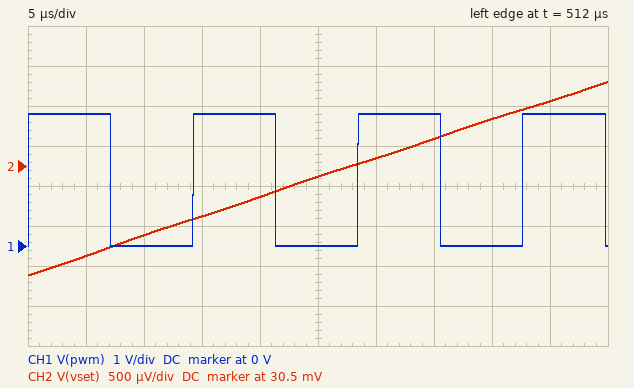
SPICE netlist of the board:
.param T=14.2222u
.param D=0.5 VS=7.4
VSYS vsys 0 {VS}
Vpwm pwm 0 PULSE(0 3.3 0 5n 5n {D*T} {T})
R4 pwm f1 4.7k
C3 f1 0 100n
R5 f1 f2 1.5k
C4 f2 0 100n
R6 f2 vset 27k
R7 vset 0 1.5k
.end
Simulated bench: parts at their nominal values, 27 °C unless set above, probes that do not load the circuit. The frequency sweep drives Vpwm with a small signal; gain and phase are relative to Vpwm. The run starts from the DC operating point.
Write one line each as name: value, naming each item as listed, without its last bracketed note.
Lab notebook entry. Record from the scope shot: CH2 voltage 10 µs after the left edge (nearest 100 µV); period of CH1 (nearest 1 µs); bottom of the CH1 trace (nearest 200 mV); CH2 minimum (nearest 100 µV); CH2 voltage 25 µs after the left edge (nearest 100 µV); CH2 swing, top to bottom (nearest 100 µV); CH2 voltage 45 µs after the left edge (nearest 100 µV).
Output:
CH2 voltage 10 µs after the left edge: 29.6 mV
period of CH1: 14 µs
bottom of the CH1 trace: 0 V
CH2 minimum: 29.1 mV
CH2 voltage 25 µs after the left edge: 30.4 mV
CH2 swing, top to bottom: 2.4 mV
CH2 voltage 45 µs after the left edge: 31.3 mV
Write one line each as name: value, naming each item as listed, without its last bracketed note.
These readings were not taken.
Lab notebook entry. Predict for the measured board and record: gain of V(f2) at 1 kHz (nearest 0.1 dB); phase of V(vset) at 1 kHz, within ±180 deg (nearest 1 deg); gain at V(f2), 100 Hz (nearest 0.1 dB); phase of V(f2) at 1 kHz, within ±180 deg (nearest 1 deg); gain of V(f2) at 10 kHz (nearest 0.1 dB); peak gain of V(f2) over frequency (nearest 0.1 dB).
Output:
gain of V(f2) at 1 kHz: -17.1 dB
phase of V(vset) at 1 kHz, within ±180 deg: -103 deg
gain at V(f2), 100 Hz: -2.8 dB
phase of V(f2) at 1 kHz, within ±180 deg: -103 deg
gain of V(f2) at 10 kHz: -49.1 dB
peak gain of V(f2) over frequency: -1.7 dB
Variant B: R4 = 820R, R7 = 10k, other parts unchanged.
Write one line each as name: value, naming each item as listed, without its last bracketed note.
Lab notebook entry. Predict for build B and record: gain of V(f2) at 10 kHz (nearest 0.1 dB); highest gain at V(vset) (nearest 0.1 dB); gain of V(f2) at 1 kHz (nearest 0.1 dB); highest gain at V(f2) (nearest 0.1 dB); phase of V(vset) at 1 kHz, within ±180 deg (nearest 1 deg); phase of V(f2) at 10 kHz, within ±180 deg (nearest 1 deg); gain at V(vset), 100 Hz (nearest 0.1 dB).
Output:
gain of V(f2) at 10 kHz: -34.2 dB
highest gain at V(vset): -11.9 dB
gain of V(f2) at 1 kHz: -6.3 dB
highest gain at V(f2): -0.5 dB
phase of V(vset) at 1 kHz, within ±180 deg: -74 deg
phase of V(f2) at 10 kHz, within ±180 deg: -157 deg
gain at V(vset), 100 Hz: -12.0 dB
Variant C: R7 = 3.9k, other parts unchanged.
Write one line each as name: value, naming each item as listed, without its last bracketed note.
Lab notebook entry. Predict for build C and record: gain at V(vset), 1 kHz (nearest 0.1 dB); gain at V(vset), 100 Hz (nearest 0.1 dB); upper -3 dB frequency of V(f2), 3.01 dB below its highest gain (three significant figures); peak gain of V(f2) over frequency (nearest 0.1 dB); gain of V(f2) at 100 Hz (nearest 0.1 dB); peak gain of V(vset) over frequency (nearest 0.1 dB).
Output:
gain at V(vset), 1 kHz: -35.1 dB
gain at V(vset), 100 Hz: -20.7 dB
upper -3 dB frequency of V(f2), 3.01 dB below its highest gain: 184 Hz
peak gain of V(f2) over frequency: -1.6 dB
gain of V(f2) at 100 Hz: -2.7 dB
peak gain of V(vset) over frequency: -19.6 dB
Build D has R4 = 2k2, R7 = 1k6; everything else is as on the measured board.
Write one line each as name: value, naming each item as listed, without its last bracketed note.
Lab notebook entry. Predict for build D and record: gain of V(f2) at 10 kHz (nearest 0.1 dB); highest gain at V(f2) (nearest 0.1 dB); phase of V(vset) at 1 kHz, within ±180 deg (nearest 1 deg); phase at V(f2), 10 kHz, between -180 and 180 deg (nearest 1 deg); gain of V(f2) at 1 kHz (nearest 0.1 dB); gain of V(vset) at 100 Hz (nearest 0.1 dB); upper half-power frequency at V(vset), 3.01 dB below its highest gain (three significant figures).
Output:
gain of V(f2) at 10 kHz: -42.6 dB
highest gain at V(f2): -1.1 dB
phase of V(vset) at 1 kHz, within ±180 deg: -93 deg
phase at V(f2), 10 kHz, between -180 and 180 deg: -164 deg
gain of V(f2) at 1 kHz: -11.6 dB
gain of V(vset) at 100 Hz: -26.5 dB
upper half-power frequency at V(vset), 3.01 dB below its highest gain: 333 Hz
